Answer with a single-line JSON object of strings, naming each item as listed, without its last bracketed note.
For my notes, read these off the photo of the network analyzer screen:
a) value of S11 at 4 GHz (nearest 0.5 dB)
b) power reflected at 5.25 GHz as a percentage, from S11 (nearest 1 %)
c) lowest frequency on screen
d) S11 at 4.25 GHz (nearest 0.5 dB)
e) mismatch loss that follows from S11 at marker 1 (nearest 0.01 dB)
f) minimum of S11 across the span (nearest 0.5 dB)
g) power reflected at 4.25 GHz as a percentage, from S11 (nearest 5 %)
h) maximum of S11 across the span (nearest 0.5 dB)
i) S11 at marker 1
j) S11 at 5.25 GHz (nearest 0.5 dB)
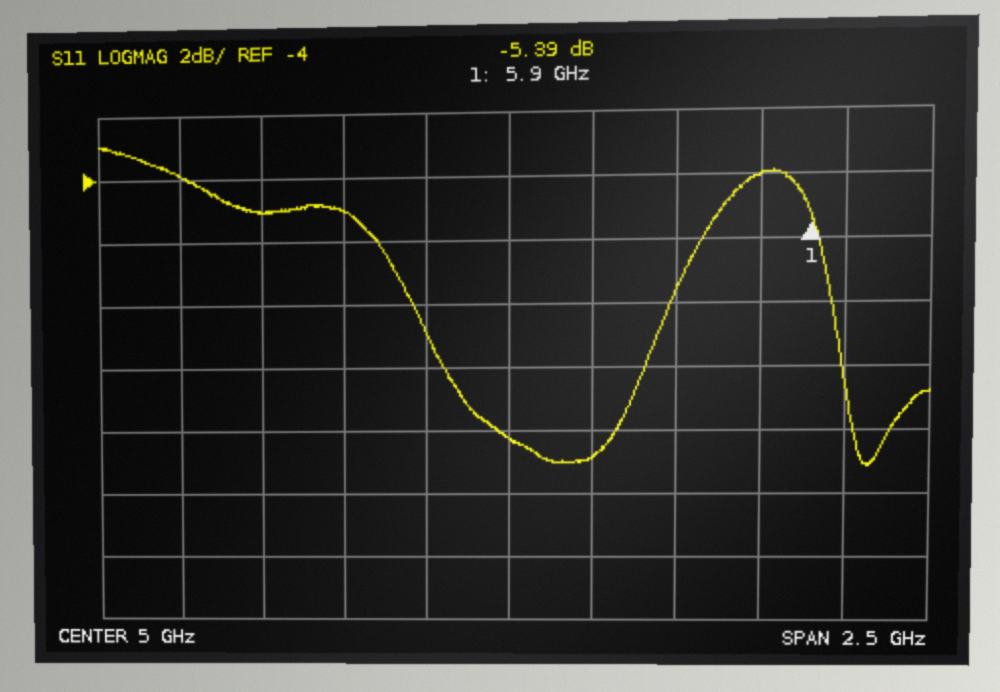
{"value of S11 at 4 GHz": "-4.0 dB", "power reflected at 5.25 GHz as a percentage, from S11": "5 %", "lowest frequency on screen": "3.75 GHz", "S11 at 4.25 GHz": "-5.0 dB", "mismatch loss that follows from S11 at marker 1": "1.48 dB", "minimum of S11 across the span": "-13.0 dB", "power reflected at 4.25 GHz as a percentage, from S11": "30 %", "maximum of S11 across the span": "-3.0 dB", "S11 at marker 1": "-5.39 dB", "S11 at 5.25 GHz": "-13.0 dB"}
